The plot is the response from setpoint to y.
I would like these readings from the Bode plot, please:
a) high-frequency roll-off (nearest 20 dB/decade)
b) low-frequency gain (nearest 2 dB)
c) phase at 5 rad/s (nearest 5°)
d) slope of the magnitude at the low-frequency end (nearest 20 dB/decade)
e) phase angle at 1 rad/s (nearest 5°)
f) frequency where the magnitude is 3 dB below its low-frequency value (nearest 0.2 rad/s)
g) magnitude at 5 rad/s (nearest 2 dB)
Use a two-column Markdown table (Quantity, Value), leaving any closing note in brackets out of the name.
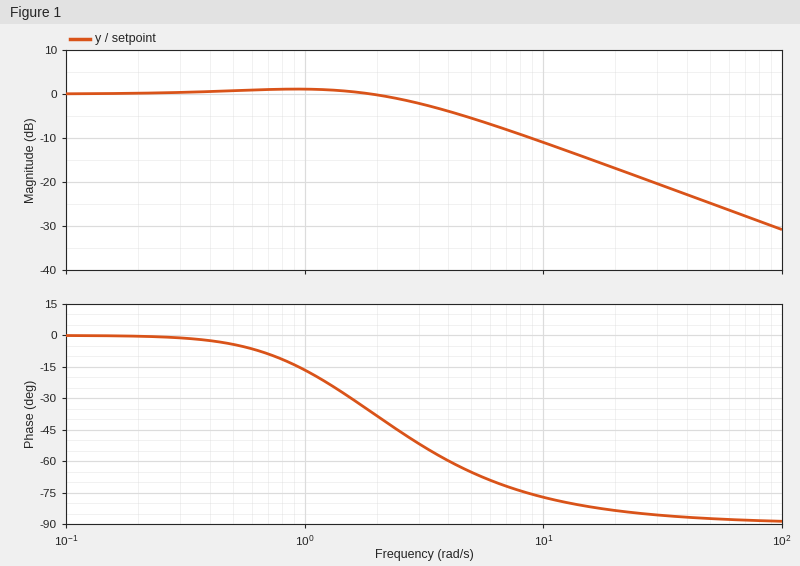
| Quantity | Value |
|---|---|
| high-frequency roll-off | -20 dB/decade |
| low-frequency gain | 0 dB |
| phase at 5 rad/s | -65° |
| slope of the magnitude at the low-frequency end | 0 dB/decade |
| phase angle at 1 rad/s | -15° |
| frequency where the magnitude is 3 dB below its low-frequency value | 3.4 rad/s |
| magnitude at 5 rad/s | -6 dB |
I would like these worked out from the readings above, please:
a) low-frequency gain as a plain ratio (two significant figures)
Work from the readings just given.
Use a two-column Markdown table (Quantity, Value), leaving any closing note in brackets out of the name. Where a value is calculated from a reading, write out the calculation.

| Quantity | Value |
|---|---|
| low-frequency gain as a plain ratio | 10^(0 / 20) = 1.0 |
